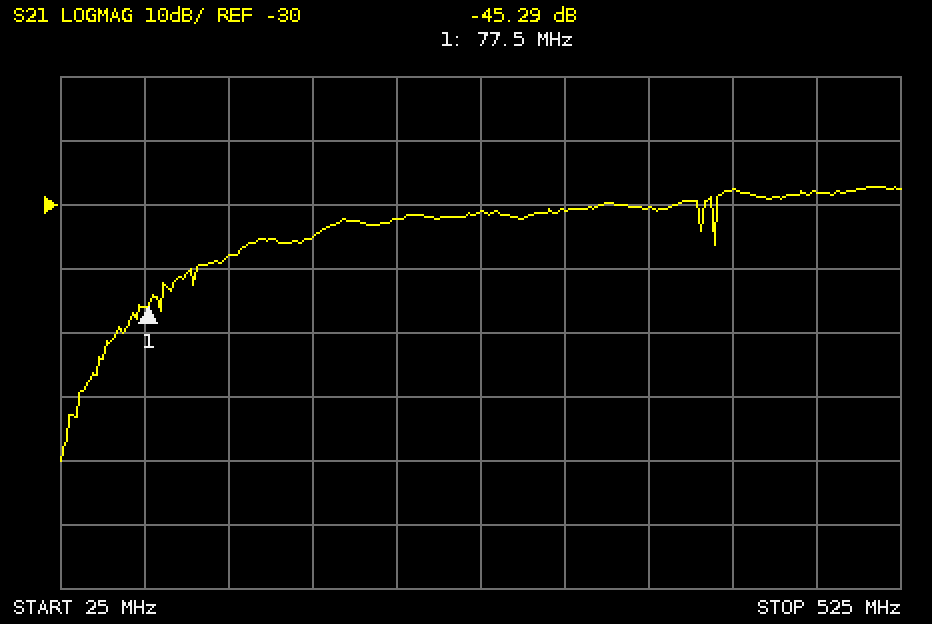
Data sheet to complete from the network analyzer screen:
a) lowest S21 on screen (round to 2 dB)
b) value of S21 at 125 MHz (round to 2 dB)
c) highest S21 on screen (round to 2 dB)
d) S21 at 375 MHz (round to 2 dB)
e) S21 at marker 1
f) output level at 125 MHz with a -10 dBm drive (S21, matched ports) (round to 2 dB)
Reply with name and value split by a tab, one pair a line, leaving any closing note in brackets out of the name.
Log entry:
lowest S21 on screen	-70 dB
value of S21 at 125 MHz	-38 dB
highest S21 on screen	-28 dB
S21 at 375 MHz	-30 dB
S21 at marker 1	-45.29 dB
output level at 125 MHz with a -10 dBm drive (S21, matched ports)	-48 dBm
